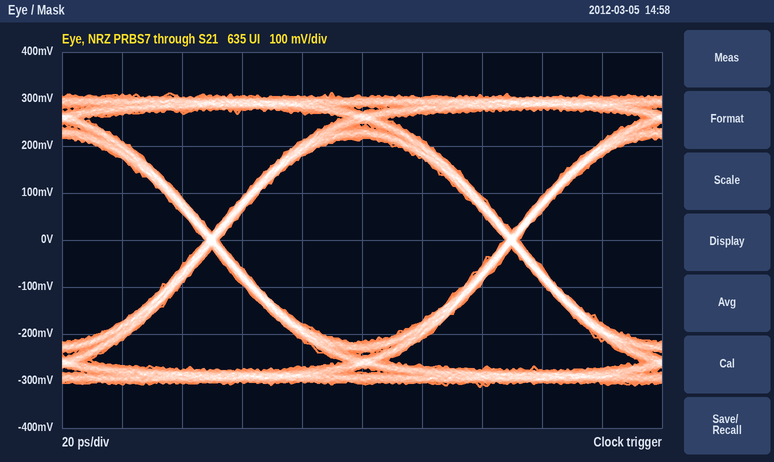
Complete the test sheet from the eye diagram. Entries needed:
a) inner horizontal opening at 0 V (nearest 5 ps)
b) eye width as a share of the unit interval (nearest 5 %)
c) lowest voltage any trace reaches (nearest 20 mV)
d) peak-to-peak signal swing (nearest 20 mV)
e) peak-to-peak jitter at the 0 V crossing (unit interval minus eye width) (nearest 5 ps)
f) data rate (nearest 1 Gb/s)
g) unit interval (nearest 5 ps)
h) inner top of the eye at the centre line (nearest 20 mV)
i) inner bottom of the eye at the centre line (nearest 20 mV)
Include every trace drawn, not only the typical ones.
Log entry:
95 ps
95 %
-320 mV
620 mV
5 ps
10 Gb/s
100 ps
220 mV
-220 mV
